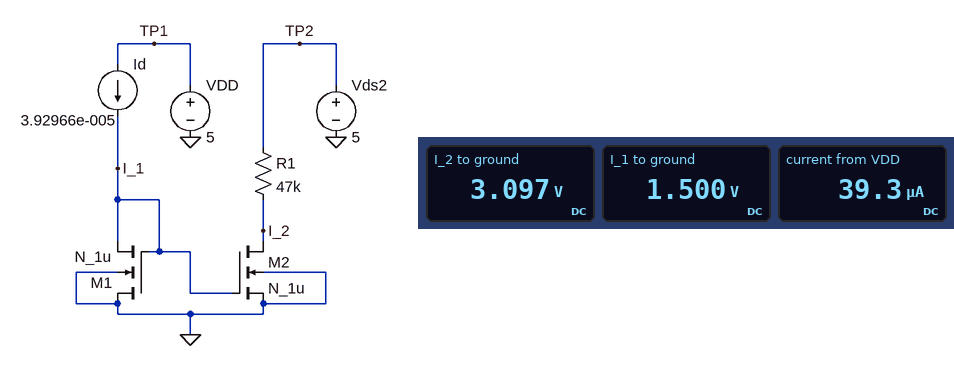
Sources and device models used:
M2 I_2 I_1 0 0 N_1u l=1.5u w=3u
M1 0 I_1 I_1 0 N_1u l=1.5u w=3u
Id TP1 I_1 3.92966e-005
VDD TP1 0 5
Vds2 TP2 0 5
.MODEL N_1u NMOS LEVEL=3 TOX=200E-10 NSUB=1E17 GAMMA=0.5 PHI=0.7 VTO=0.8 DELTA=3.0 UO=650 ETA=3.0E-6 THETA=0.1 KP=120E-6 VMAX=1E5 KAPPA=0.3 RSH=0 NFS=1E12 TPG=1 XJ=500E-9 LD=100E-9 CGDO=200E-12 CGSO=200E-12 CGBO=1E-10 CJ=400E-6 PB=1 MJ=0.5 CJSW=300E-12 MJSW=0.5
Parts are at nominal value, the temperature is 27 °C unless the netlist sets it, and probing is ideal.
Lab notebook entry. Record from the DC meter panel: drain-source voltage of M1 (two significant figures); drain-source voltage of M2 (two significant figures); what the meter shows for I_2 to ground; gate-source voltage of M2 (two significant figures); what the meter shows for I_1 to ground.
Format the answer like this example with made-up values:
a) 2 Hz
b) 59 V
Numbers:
a) -1.5 V
b) 3.1 V
c) 3.097 V
d) 1.5 V
e) 1.500 V
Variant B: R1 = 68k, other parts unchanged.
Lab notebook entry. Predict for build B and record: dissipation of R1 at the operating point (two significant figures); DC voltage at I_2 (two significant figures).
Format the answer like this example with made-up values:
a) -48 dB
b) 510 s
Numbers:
a) 110 µW
b) 2.3 V
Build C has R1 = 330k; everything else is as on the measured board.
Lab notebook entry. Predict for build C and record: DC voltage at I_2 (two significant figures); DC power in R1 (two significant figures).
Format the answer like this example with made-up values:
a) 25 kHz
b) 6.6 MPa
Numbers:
a) 99 mV
b) 73 µW
